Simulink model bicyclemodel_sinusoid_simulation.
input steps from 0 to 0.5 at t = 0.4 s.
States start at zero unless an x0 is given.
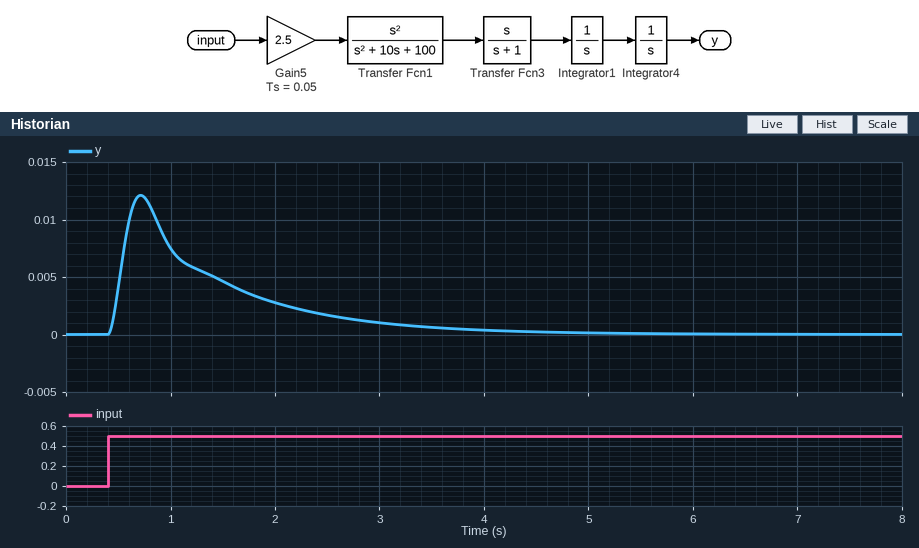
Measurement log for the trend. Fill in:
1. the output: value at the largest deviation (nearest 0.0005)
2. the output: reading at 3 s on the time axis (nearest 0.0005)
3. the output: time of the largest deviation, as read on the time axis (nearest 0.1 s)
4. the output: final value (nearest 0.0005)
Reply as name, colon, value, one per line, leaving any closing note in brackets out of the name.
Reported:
the output: value at the largest deviation: 0.0120
the output: reading at 3 s on the time axis: 0.0010
the output: time of the largest deviation, as read on the time axis: 0.7 s
the output: final value: 0.0000
